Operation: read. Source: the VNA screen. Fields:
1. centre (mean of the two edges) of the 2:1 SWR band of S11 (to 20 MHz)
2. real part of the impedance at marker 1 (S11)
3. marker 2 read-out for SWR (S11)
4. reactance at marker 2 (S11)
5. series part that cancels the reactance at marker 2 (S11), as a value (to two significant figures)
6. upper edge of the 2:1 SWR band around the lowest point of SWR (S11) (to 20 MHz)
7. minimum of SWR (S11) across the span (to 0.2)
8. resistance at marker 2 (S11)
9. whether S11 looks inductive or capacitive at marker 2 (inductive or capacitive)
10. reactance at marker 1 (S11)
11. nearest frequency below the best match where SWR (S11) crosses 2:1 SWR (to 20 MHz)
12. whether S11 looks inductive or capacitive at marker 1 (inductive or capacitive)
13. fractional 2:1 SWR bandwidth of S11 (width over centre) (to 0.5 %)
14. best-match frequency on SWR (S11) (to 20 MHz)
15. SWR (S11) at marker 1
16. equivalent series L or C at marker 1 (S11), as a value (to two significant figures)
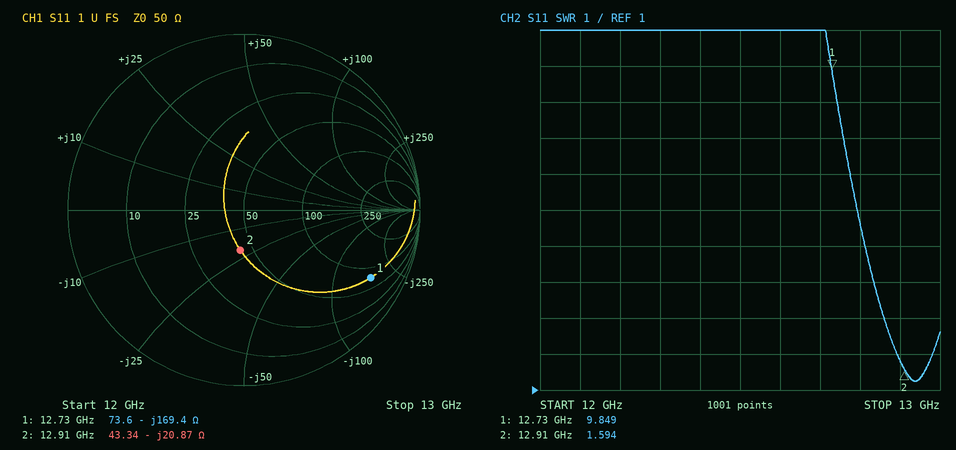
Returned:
12.94 GHz
73.6 Ω
1.594
-20.87 Ω
260 pH
12.98 GHz
1.2
43.34 Ω
capacitive
-169.4 Ω
12.90 GHz
capacitive
0.5 %
12.94 GHz
9.849
74 fF
